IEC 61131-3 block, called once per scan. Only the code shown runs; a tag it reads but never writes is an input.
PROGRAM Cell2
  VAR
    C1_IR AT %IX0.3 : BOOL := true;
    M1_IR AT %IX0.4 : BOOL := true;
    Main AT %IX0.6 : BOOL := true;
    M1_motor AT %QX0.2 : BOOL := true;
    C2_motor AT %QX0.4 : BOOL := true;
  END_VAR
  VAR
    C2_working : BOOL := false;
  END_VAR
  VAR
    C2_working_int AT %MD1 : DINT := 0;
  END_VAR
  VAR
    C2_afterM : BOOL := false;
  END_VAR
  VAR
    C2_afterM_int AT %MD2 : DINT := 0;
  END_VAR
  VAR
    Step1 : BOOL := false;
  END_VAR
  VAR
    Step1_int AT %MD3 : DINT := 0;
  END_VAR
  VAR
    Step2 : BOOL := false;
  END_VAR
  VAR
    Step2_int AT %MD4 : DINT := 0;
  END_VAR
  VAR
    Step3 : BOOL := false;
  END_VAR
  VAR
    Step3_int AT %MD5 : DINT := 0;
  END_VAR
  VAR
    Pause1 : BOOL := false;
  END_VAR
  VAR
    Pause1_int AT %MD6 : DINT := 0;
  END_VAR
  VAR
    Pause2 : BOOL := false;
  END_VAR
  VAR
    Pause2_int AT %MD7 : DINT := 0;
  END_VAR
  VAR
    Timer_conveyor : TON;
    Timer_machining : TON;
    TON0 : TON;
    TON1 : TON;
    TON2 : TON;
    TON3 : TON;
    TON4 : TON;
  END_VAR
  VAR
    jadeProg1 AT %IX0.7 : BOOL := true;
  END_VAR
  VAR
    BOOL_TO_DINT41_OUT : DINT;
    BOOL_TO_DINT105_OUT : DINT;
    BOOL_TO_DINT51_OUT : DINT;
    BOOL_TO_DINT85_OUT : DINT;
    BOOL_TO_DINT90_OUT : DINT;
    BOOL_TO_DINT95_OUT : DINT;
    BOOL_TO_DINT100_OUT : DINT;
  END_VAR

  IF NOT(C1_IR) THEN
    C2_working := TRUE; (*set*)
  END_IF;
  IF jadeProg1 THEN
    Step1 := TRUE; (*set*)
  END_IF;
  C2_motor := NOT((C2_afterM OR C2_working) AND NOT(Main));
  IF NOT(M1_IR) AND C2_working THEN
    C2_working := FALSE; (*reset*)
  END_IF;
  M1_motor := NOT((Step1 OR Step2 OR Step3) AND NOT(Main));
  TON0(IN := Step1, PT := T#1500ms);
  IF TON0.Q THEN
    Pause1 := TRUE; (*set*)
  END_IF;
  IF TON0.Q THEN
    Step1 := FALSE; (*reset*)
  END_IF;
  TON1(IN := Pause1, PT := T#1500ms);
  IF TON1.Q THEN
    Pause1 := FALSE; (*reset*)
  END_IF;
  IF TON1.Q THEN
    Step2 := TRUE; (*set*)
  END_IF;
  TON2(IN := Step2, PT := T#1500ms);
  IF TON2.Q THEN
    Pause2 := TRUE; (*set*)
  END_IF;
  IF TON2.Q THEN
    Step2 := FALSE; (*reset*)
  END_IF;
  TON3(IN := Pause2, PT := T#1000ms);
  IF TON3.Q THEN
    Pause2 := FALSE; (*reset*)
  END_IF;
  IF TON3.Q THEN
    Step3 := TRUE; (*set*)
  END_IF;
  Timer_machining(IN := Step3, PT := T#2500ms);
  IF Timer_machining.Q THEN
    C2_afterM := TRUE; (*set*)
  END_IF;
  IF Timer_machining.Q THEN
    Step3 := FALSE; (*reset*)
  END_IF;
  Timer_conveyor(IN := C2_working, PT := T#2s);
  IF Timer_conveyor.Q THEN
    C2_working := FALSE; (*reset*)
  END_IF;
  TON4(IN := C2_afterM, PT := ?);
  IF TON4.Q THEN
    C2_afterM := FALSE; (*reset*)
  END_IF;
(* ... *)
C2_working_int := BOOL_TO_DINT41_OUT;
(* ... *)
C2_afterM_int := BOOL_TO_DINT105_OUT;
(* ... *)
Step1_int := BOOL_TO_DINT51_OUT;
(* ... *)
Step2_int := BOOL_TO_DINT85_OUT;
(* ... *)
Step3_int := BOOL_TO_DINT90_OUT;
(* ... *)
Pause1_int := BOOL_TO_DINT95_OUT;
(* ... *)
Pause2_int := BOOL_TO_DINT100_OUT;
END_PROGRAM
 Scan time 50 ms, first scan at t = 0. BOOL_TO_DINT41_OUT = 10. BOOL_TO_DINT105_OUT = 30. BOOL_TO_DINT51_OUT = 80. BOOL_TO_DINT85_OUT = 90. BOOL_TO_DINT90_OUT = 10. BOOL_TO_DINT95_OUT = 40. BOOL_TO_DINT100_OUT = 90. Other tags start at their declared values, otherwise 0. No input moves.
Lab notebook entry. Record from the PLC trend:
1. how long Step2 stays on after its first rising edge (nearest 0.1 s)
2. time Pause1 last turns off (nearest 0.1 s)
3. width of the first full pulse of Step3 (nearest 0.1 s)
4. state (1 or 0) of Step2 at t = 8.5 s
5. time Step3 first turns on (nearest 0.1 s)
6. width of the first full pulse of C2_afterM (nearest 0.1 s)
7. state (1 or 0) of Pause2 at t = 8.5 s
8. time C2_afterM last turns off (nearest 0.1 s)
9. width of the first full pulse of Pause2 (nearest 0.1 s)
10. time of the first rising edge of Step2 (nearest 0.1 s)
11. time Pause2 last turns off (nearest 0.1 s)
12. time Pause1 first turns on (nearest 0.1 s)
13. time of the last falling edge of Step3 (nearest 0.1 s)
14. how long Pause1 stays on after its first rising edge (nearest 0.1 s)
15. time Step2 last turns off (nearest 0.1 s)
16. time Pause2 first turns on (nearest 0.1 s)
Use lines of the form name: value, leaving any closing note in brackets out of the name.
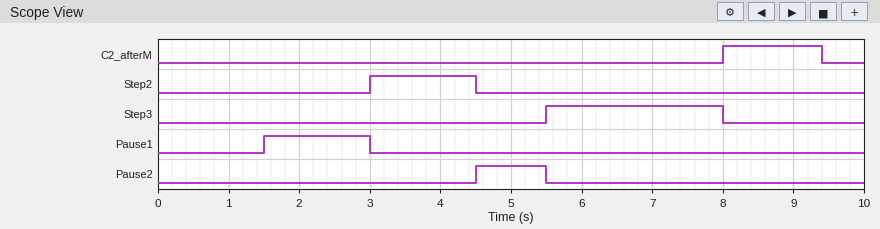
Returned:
how long Step2 stays on after its first rising edge: 1.5 s
time Pause1 last turns off: 3.0 s
width of the first full pulse of Step3: 2.5 s
state (1 or 0) of Step2 at t = 8.5 s: 0
time Step3 first turns on: 5.5 s
width of the first full pulse of C2_afterM: 1.4 s
state (1 or 0) of Pause2 at t = 8.5 s: 0
time C2_afterM last turns off: 9.4 s
width of the first full pulse of Pause2: 1.0 s
time of the first rising edge of Step2: 3.0 s
time Pause2 last turns off: 5.5 s
time Pause1 first turns on: 1.5 s
time of the last falling edge of Step3: 8.0 s
how long Pause1 stays on after its first rising edge: 1.5 s
time Step2 last turns off: 4.5 s
time Pause2 first turns on: 4.5 s
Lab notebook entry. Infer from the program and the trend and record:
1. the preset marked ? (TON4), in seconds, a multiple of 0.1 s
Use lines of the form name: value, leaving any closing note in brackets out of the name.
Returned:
the preset marked ? (TON4), in seconds, a multiple of 0.1 s: 1.4 s
